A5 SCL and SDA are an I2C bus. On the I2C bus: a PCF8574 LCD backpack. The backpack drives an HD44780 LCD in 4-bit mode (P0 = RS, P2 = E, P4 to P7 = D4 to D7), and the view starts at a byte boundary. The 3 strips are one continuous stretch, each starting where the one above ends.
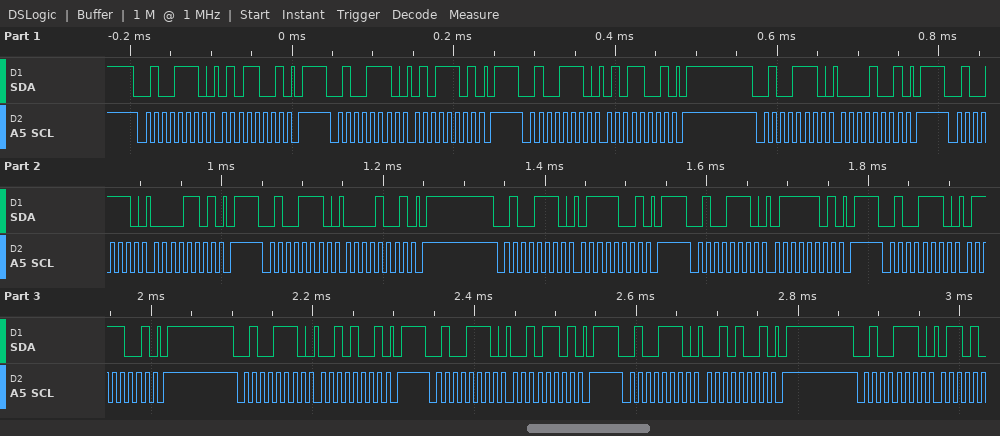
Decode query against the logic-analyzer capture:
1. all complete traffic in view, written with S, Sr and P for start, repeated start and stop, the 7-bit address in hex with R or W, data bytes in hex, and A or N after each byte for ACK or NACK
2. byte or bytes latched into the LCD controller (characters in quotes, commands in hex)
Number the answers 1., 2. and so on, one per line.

1. S 27W A 59 A P S 27W A 5D A P S 27W A 59 A P S 27W A 09 A P S 27W A 0D A P S 27W A 09 A P S 27W A 79 A P S 27W A 7D A P S 27W A 79 A P S 27W A 29 A P S 27W A 2D A P S 27W A 29 A P S 27W A
2. 'P' 'r'
